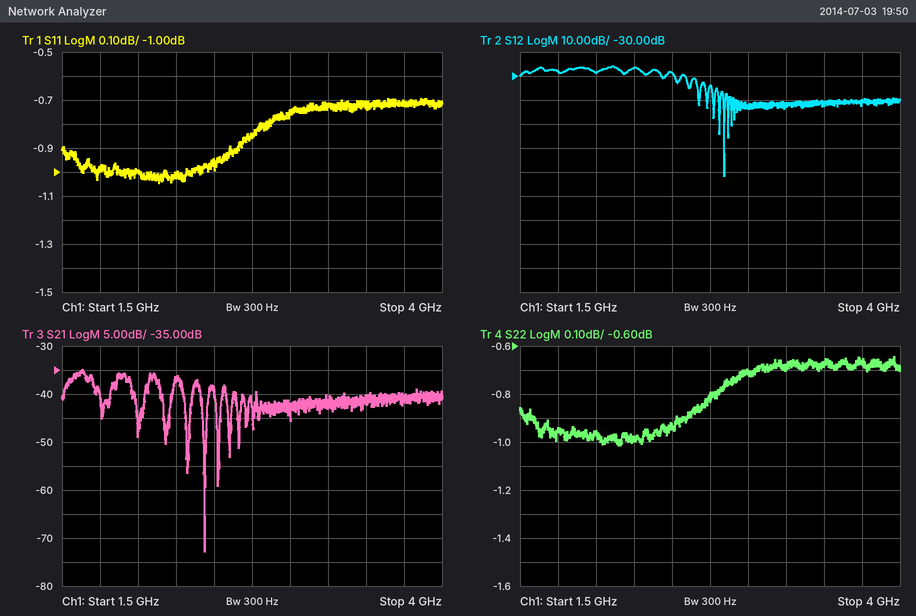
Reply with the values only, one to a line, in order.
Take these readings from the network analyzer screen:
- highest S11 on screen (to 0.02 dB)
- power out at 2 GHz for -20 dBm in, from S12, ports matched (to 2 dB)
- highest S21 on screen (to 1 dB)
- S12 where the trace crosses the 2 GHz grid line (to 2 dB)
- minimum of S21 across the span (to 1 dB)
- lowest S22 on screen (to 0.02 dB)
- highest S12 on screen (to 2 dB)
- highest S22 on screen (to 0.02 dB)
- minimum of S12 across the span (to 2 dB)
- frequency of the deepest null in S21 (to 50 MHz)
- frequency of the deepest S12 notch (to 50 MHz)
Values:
-0.70 dB
-48 dBm
-35 dB
-28 dB
-73 dB
-1.02 dB
-26 dB
-0.64 dB
-72 dB
2.45 GHz
2.85 GHz
